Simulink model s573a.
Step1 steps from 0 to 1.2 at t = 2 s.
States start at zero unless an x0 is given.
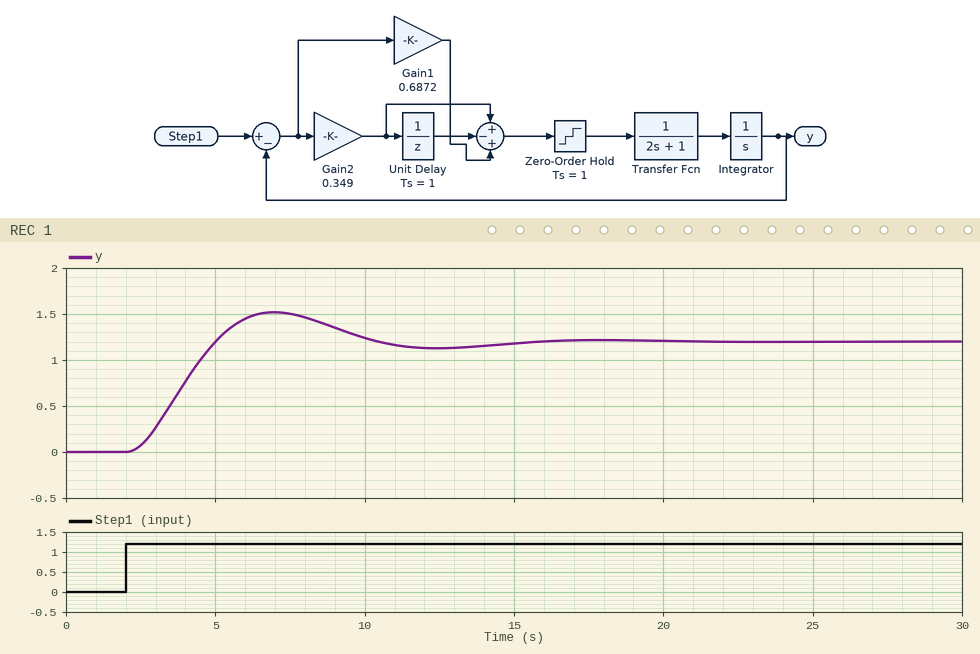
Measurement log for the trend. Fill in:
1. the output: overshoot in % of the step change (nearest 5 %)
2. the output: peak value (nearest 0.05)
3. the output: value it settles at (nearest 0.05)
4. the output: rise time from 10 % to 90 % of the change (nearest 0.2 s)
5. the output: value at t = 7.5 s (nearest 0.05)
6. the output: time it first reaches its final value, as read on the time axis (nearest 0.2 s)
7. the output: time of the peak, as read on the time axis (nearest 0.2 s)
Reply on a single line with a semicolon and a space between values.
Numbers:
25 %; 1.50; 1.20; 2.0 s; 1.50; 5.0 s; 7.0 s
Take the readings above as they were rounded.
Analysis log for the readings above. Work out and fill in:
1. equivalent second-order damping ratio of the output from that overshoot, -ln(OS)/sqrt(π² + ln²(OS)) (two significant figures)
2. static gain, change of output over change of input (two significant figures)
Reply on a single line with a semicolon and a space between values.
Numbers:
0.40; 1.0
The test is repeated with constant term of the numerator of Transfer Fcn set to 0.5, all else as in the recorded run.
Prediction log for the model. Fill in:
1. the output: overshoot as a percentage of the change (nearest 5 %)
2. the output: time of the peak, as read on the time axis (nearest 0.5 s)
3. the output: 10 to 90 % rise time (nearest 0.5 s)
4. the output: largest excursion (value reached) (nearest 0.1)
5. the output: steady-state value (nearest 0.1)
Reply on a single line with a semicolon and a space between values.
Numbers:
10 %; 10.5 s; 4.0 s; 1.3; 1.2
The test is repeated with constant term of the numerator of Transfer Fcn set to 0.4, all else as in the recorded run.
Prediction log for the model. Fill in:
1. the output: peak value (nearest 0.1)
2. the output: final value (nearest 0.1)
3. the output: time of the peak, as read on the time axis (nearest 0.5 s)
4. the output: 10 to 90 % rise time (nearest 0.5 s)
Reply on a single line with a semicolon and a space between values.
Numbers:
1.3; 1.2; 12.5 s; 5.0 s
